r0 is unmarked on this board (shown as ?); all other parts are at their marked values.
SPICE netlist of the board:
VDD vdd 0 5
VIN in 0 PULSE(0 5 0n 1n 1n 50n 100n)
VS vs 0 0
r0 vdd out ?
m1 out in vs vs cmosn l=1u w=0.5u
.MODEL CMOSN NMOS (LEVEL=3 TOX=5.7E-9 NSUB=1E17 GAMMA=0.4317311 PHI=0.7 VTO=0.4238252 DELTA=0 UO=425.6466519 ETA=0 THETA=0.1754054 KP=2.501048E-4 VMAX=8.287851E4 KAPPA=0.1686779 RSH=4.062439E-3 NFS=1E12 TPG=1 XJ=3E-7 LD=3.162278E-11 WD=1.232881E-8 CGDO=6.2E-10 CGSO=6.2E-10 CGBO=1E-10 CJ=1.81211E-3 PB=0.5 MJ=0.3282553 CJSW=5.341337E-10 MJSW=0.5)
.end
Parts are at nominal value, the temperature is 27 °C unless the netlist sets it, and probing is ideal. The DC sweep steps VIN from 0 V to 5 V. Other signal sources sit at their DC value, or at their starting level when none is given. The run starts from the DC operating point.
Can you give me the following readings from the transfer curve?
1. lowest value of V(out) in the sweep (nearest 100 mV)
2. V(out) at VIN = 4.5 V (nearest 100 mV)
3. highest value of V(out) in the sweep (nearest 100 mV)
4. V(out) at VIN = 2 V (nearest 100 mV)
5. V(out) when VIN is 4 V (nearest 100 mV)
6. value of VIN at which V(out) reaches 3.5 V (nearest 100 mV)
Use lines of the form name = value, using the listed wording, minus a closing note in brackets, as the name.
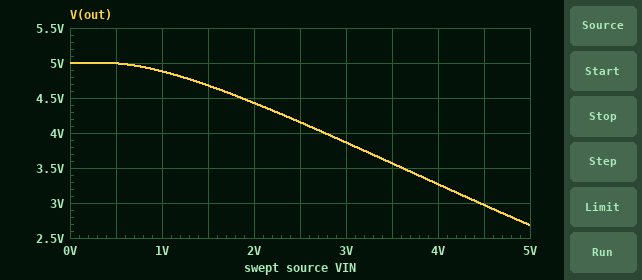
lowest value of V(out) in the sweep = 2.7 V
V(out) at VIN = 4.5 V = 3.0 V
highest value of V(out) in the sweep = 5.0 V
V(out) at VIN = 2 V = 4.4 V
V(out) when VIN is 4 V = 3.3 V
value of VIN at which V(out) reaches 3.5 V = 3.6 V
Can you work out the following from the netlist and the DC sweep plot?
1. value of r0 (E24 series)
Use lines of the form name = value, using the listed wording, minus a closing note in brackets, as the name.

value of r0 = 7.5 kΩ
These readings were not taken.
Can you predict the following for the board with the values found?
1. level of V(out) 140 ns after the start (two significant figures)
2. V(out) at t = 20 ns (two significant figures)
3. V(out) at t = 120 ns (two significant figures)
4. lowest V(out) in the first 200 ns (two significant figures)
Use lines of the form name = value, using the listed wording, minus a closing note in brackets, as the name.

level of V(out) 140 ns after the start = 2.7 V
V(out) at t = 20 ns = 2.7 V
V(out) at t = 120 ns = 2.7 V
lowest V(out) in the first 200 ns = 2.7 V
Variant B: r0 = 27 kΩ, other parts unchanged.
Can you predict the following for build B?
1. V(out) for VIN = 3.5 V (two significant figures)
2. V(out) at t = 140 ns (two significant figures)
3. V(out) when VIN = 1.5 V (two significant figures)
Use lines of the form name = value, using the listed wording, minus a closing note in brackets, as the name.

V(out) for VIN = 3.5 V = 1.0 V
V(out) at t = 140 ns = 690 mV
V(out) when VIN = 1.5 V = 3.9 V
